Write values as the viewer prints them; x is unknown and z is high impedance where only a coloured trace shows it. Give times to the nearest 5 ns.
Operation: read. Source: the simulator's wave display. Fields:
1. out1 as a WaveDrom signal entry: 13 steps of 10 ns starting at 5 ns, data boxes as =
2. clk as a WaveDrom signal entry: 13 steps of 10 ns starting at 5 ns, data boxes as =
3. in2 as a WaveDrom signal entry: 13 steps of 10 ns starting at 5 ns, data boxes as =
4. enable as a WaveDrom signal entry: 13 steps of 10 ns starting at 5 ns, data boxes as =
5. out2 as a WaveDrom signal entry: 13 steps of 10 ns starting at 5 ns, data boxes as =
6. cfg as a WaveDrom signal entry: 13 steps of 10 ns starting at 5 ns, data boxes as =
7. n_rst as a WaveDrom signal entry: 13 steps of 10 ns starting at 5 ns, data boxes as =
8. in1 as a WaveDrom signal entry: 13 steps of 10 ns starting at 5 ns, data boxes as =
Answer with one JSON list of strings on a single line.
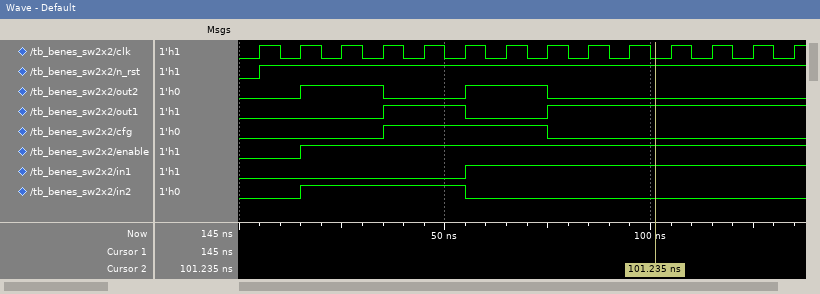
["{name: 'out1', wave: '0..1.0.1.....'}", "{name: 'clk', wave: 'p............'}", "{name: 'in2', wave: '01...0.......'}", "{name: 'enable', wave: '01...........'}", "{name: 'out2', wave: '01.0.1.0.....'}", "{name: 'cfg', wave: '0..1...0.....'}", "{name: 'n_rst', wave: '1............'}", "{name: 'in1', wave: '0....1.......'}"]
